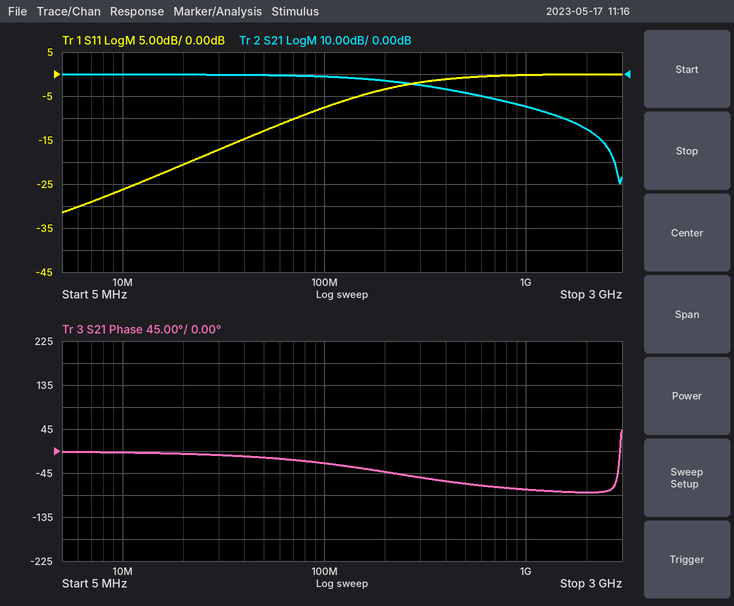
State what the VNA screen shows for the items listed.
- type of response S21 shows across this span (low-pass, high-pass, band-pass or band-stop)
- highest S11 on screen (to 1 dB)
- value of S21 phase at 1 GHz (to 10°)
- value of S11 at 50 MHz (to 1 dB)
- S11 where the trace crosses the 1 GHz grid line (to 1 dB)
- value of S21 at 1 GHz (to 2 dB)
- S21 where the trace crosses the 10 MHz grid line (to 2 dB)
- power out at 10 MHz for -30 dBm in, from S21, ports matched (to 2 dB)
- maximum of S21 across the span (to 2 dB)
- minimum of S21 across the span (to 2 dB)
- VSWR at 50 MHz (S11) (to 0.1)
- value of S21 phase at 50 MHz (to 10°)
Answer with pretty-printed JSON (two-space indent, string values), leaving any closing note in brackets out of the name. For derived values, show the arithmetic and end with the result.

{
  "type of response S21 shows across this span": "low-pass",
  "highest S11 on screen": "0 dB",
  "value of S21 phase at 1 GHz": "-80°",
  "value of S11 at 50 MHz": "-13 dB",
  "S11 where the trace crosses the 1 GHz grid line": "0 dB",
  "value of S21 at 1 GHz": "-14 dB",
  "S21 where the trace crosses the 10 MHz grid line": "0 dB",
  "power out at 10 MHz for -30 dBm in, from S21, ports matched": "-30 dBm + (0 dB) = -30 dBm",
  "maximum of S21 across the span": "0 dB",
  "minimum of S21 across the span": "-50 dB",
  "VSWR at 50 MHz (S11)": "|Γ| = 10^(-13/20) = 0.2239; VSWR = (1 + 0.2239)/(1 − 0.2239) ≈ 1.6",
  "value of S21 phase at 50 MHz": "-10°"
}
